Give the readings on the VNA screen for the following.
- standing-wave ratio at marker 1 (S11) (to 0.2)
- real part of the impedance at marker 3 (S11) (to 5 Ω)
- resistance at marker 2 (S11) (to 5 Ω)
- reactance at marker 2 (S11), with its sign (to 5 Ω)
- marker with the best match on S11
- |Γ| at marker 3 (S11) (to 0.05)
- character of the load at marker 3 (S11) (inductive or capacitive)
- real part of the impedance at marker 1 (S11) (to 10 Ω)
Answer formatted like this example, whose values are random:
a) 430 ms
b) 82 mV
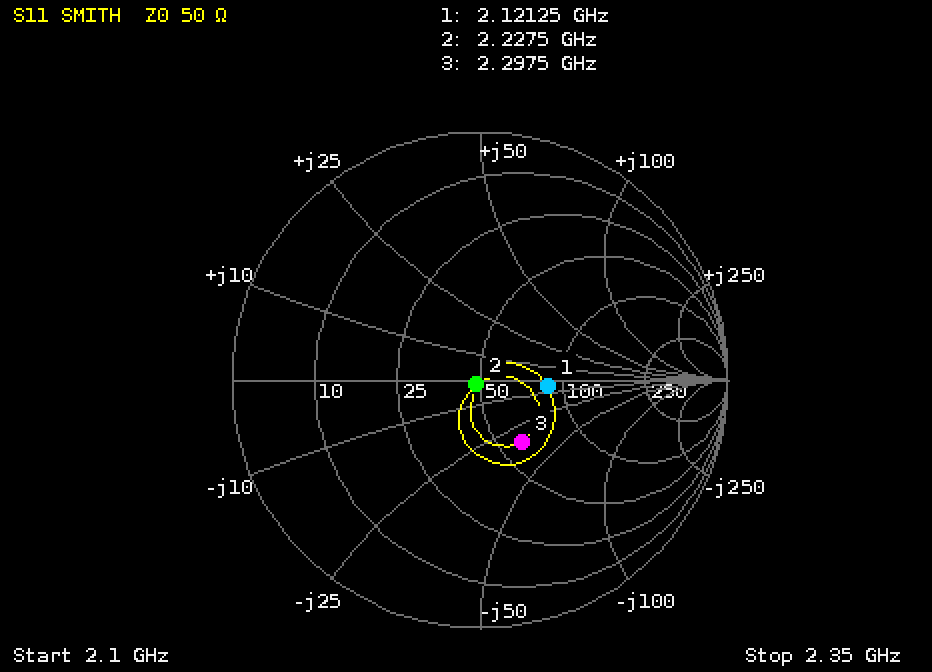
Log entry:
a) 1.8
b) 60 Ω
c) 50 Ω
d) 0 Ω
e) marker 2
f) 0.30
g) capacitive
h) 90 Ω
